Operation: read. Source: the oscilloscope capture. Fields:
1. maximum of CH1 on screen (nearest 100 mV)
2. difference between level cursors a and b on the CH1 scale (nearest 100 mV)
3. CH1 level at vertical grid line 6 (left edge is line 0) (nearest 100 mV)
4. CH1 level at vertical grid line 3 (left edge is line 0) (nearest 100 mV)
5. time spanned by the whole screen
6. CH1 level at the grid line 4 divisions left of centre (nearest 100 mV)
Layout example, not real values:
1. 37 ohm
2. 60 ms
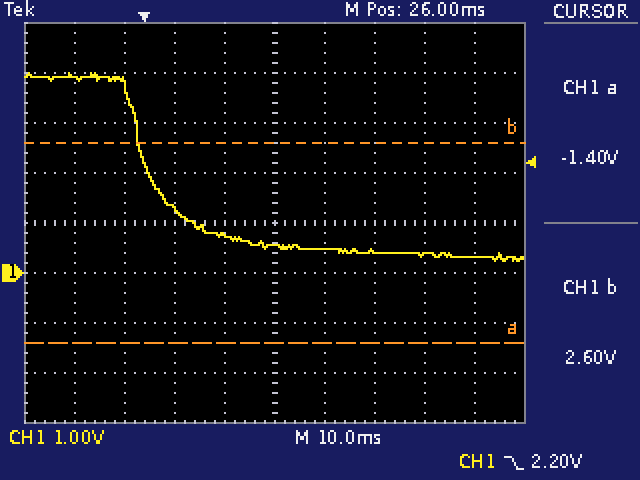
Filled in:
1. 4.0 V
2. 4.0 V
3. 500 mV
4. 1.3 V
5. 100 ms
6. 3.9 V
